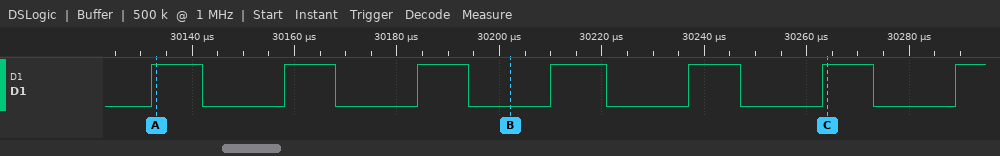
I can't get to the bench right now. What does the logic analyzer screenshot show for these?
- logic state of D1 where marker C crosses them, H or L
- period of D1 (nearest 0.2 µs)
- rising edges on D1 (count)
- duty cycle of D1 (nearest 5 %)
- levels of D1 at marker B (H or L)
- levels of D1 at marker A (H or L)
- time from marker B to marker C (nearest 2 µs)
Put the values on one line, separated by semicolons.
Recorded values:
D1=H; 26.2 µs; 7; 40 %; D1=L; D1=H; 62 µs
